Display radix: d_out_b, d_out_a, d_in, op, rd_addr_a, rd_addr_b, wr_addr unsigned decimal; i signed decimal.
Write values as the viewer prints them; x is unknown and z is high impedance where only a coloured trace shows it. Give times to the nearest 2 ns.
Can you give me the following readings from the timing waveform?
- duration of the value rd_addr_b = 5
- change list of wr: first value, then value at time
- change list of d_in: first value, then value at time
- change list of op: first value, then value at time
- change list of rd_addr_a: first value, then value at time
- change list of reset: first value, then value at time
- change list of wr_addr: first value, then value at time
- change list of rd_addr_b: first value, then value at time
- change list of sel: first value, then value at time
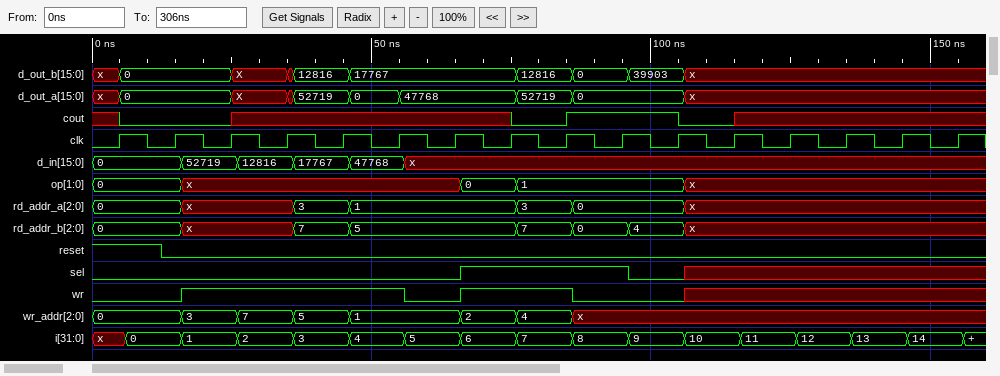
30 ns
0, 1 at 16 ns, 0 at 56 ns, 1 at 66 ns, 0 at 86 ns, x at 106 ns
0, 52719 at 16 ns, 12816 at 26 ns, 17767 at 36 ns, 47768 at 46 ns, x at 56 ns
0, x at 16 ns, 0 at 66 ns, 1 at 76 ns, x at 106 ns
0, x at 16 ns, 3 at 36 ns, 1 at 46 ns, 3 at 76 ns, 0 at 86 ns, x at 106 ns
1, 0 at 12 ns
0, 3 at 16 ns, 7 at 26 ns, 5 at 36 ns, 1 at 46 ns, 2 at 66 ns, 4 at 76 ns, x at 86 ns
0, x at 16 ns, 7 at 36 ns, 5 at 46 ns, 7 at 76 ns, 0 at 86 ns, 4 at 96 ns, x at 106 ns
0, 1 at 66 ns, 0 at 96 ns, x at 106 ns
